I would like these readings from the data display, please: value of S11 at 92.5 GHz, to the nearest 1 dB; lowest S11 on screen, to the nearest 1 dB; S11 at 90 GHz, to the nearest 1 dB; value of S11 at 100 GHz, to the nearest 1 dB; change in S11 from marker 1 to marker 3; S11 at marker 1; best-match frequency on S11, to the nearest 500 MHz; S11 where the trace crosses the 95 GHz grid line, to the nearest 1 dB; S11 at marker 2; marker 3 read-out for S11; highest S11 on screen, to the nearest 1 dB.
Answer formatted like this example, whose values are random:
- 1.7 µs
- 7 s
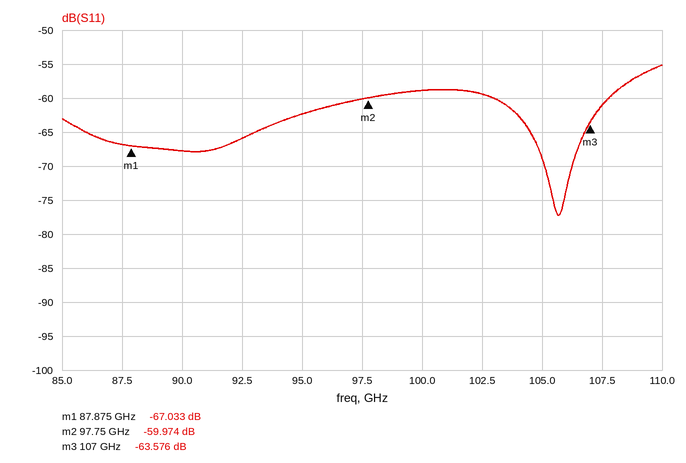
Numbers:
- -66 dB
- -77 dB
- -68 dB
- -59 dB
- 3.457 dB
- -67.033 dB
- 105.5 GHz
- -62 dB
- -59.974 dB
- -63.576 dB
- -55 dB
